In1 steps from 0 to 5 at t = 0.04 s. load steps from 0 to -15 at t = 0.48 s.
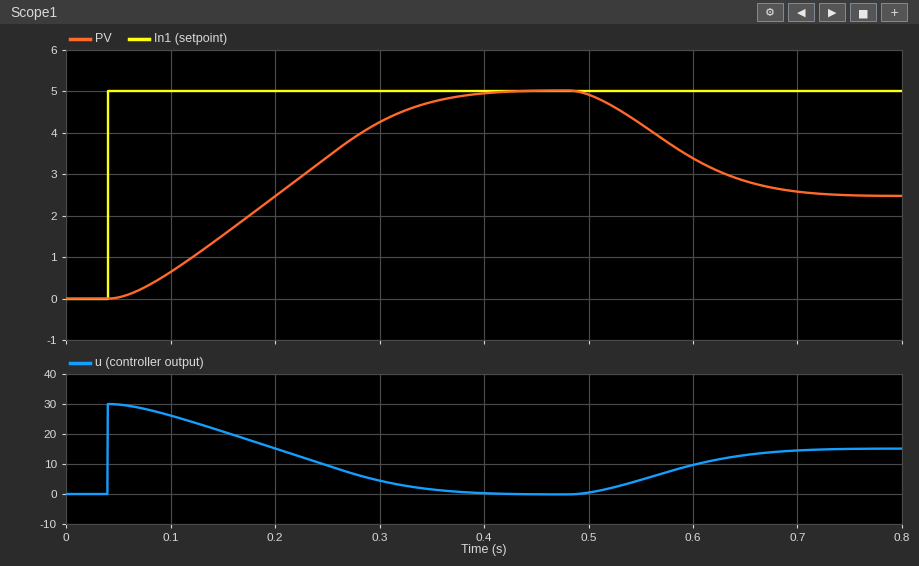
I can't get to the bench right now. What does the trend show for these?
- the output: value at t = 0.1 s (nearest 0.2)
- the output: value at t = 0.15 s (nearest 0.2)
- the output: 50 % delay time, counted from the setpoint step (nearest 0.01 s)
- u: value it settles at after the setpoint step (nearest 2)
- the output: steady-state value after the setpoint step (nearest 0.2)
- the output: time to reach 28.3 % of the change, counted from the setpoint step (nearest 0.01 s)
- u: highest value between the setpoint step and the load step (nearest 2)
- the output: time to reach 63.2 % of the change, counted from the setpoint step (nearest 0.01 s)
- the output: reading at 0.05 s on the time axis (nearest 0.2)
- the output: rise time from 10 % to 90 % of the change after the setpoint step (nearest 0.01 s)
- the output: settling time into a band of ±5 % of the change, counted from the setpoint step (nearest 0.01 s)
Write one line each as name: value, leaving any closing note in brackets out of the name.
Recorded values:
the output: value at t = 0.1 s: 0.6
the output: value at t = 0.15 s: 1.6
the output: 50 % delay time, counted from the setpoint step: 0.16 s
u: value it settles at after the setpoint step: 0
the output: steady-state value after the setpoint step: 5.0
the output: time to reach 28.3 % of the change, counted from the setpoint step: 0.10 s
u: highest value between the setpoint step and the load step: 30
the output: time to reach 63.2 % of the change, counted from the setpoint step: 0.20 s
the output: reading at 0.05 s on the time axis: 0.0
the output: rise time from 10 % to 90 % of the change after the setpoint step: 0.23 s
the output: settling time into a band of ±5 % of the change, counted from the setpoint step: 0.31 s
